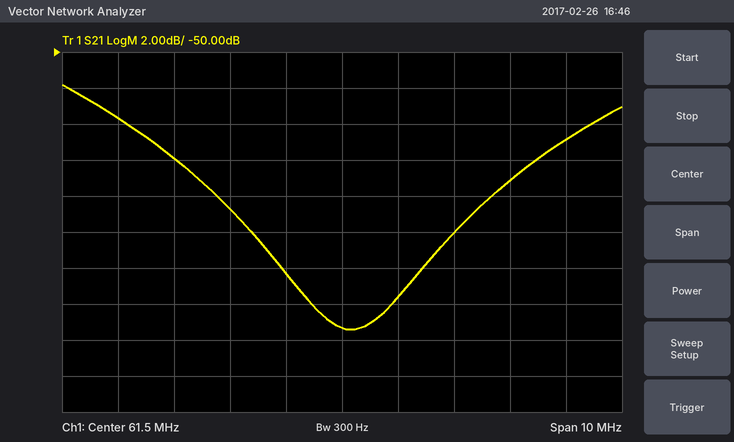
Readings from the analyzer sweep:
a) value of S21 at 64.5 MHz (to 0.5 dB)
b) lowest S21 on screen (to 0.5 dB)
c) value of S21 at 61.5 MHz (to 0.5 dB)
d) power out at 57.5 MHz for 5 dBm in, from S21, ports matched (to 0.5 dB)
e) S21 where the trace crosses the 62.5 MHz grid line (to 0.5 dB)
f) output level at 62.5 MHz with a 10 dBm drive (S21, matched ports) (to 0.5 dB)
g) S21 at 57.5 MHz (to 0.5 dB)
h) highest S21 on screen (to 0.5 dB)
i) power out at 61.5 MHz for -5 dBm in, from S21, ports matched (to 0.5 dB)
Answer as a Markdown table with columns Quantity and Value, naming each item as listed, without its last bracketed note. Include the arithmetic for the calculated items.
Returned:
| Quantity | Value |
|---|---|
| value of S21 at 64.5 MHz | -57.0 dB |
| lowest S21 on screen | -65.5 dB |
| value of S21 at 61.5 MHz | -65.5 dB |
| power out at 57.5 MHz for 5 dBm in, from S21, ports matched | 5 dBm + (-53.5 dB) = -48.5 dBm |
| S21 where the trace crosses the 62.5 MHz grid line | -63.5 dB |
| output level at 62.5 MHz with a 10 dBm drive (S21, matched ports) | 10 dBm + (-63.5 dB) = -53.5 dBm |
| S21 at 57.5 MHz | -53.5 dB |
| highest S21 on screen | -52.0 dB |
| power out at 61.5 MHz for -5 dBm in, from S21, ports matched | -5 dBm + (-65.5 dB) = -70.5 dBm |
